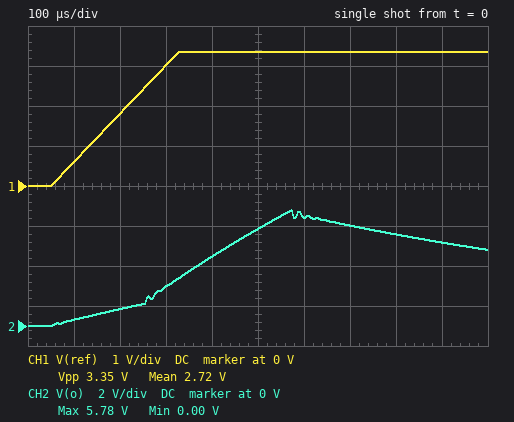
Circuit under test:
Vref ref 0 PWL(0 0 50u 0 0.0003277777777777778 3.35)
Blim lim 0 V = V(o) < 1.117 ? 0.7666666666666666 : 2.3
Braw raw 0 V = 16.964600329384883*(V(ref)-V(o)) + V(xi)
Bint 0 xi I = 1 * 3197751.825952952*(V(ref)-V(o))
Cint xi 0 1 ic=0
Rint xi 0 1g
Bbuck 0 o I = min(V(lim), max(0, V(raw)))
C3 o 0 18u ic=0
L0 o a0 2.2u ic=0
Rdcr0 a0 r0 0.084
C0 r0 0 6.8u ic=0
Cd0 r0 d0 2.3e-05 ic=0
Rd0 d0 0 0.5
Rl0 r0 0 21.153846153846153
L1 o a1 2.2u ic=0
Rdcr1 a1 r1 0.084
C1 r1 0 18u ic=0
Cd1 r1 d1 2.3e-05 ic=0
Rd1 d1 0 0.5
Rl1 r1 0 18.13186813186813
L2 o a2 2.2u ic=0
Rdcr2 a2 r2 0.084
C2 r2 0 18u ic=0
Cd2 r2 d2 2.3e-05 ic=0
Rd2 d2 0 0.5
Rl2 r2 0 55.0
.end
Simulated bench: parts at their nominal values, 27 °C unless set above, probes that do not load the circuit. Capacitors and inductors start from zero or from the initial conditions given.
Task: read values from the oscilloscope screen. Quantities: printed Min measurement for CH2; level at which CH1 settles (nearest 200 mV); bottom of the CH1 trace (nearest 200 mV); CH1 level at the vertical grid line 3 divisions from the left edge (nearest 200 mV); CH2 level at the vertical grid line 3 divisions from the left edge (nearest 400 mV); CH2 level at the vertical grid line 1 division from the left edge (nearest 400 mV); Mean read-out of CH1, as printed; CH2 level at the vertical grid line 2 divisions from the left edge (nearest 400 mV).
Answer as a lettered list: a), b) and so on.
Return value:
a) 0.00 V
b) 3.4 V
c) 0 V
d) 3.0 V
e) 2.0 V
f) 400 mV
g) 2.72 V
h) 800 mV
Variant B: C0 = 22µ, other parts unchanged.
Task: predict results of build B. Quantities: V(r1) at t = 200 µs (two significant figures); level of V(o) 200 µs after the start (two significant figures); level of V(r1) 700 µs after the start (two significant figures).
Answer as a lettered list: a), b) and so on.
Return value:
a) 740 mV
b) 760 mV
c) 5.7 V
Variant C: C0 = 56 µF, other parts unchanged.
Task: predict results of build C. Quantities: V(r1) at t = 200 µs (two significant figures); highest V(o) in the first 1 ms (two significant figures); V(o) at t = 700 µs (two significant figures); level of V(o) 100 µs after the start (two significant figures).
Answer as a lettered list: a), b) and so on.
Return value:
a) 610 mV
b) 6.4 V
c) 5.1 V
d) 230 mV
